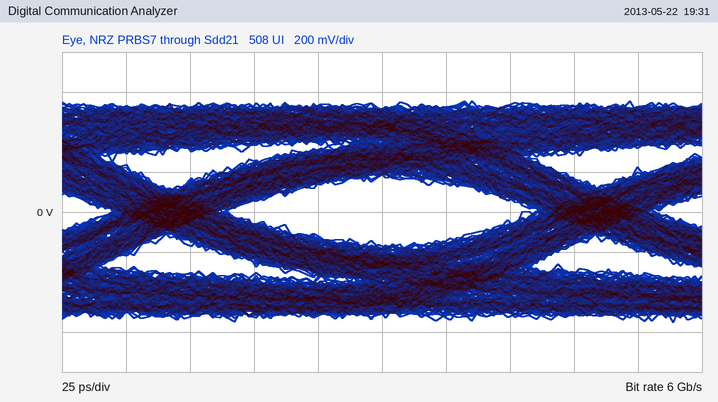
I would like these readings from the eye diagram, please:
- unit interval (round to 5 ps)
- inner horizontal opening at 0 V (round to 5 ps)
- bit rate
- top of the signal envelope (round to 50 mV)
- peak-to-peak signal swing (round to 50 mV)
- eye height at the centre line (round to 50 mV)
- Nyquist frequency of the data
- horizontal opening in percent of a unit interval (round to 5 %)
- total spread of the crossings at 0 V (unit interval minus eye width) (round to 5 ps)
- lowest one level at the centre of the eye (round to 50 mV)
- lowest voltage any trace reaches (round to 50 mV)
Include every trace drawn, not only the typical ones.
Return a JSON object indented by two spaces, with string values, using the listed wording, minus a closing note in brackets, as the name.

{
  "unit interval": "165 ps",
  "inner horizontal opening at 0 V": "115 ps",
  "bit rate": "6 Gb/s",
  "top of the signal envelope": "550 mV",
  "peak-to-peak signal swing": "1.10 V",
  "eye height at the centre line": "350 mV",
  "Nyquist frequency of the data": "3 GHz",
  "horizontal opening in percent of a unit interval": "70 %",
  "total spread of the crossings at 0 V (unit interval minus eye width)": "50 ps",
  "lowest one level at the centre of the eye": "200 mV",
  "lowest voltage any trace reaches": "-550 mV"
}
